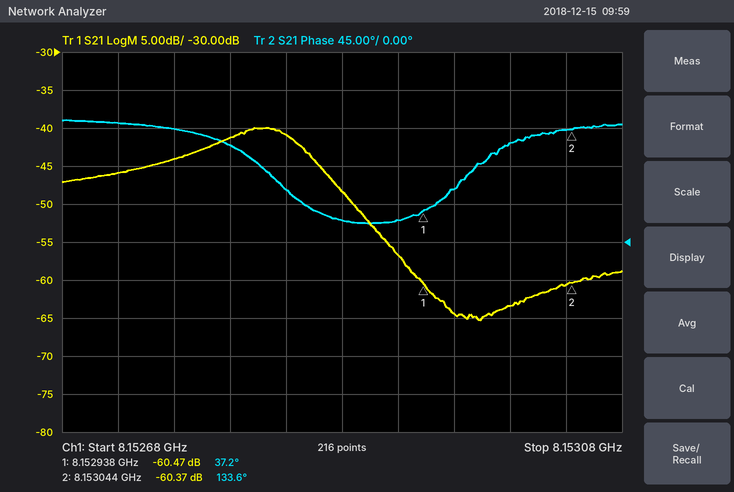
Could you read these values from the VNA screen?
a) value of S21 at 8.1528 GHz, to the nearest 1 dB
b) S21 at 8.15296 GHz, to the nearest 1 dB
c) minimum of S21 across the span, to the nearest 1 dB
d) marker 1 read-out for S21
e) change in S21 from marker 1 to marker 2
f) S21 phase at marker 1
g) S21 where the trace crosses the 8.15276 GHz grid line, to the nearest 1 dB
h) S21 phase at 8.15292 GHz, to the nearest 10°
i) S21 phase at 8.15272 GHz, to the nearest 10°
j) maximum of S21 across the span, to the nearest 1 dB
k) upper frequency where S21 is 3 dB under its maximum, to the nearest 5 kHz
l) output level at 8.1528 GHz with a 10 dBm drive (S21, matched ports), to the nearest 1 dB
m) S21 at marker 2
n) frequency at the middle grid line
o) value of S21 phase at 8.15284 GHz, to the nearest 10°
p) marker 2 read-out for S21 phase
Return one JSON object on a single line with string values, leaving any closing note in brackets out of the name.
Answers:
{"value of S21 at 8.1528 GHz, to the nearest 1 dB": "-41 dB", "S21 at 8.15296 GHz, to the nearest 1 dB": "-64 dB", "minimum of S21 across the span, to the nearest 1 dB": "-65 dB", "marker 1 read-out for S21": "-60.47 dB", "change in S21 from marker 1 to marker 2": "0.10 dB", "S21 phase at marker 1": "37.2°", "S21 where the trace crosses the 8.15276 GHz grid line, to the nearest 1 dB": "-44 dB", "S21 phase at 8.15292 GHz, to the nearest 10°": "30°", "S21 phase at 8.15272 GHz, to the nearest 10°": "140°", "maximum of S21 across the span, to the nearest 1 dB": "-40 dB", "upper frequency where S21 is 3 dB under its maximum, to the nearest 5 kHz": "8.152855 GHz", "output level at 8.1528 GHz with a 10 dBm drive (S21, matched ports), to the nearest 1 dB": "-31 dBm", "S21 at marker 2": "-60.37 dB", "frequency at the middle grid line": "8.15288 GHz", "value of S21 phase at 8.15284 GHz, to the nearest 10°": "60°", "marker 2 read-out for S21 phase": "133.6°"}
